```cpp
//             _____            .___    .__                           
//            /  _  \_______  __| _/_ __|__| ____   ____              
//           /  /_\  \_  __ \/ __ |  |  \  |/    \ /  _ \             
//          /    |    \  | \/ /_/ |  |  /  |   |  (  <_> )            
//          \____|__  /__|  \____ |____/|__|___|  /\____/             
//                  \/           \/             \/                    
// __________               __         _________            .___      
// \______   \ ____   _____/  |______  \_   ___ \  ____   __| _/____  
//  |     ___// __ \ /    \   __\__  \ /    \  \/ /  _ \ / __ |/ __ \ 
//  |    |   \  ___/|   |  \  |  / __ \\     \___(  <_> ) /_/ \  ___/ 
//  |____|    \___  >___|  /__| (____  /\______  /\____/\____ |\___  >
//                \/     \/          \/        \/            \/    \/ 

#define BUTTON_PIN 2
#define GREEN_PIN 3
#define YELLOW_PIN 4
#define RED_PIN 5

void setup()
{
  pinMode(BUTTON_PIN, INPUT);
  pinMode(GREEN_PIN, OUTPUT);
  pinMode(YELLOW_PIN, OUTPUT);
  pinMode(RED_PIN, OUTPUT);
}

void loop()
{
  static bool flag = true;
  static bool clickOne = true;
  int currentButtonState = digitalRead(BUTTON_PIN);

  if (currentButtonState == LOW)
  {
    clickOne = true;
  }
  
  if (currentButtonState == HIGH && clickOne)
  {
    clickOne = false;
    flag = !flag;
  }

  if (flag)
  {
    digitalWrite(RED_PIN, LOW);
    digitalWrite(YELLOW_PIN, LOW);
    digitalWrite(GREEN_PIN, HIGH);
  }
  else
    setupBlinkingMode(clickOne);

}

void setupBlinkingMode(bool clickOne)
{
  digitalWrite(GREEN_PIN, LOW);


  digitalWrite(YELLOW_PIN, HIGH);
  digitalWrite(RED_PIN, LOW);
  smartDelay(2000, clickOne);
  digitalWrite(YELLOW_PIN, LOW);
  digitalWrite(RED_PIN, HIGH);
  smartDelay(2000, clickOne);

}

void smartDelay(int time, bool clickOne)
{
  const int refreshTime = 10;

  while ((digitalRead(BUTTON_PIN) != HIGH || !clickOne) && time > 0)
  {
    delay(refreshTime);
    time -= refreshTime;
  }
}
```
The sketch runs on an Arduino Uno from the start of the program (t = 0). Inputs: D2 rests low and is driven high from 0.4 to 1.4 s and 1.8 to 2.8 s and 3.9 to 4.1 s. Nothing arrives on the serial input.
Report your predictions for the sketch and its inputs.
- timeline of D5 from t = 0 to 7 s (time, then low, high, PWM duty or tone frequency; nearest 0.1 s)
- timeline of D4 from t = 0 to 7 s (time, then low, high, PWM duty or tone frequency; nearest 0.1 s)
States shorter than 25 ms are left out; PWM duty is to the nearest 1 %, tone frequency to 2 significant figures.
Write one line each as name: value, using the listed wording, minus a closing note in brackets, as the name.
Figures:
timeline of D5 from t = 0 to 7 s: 0 s low; 2.4 s high; 4.4 s low; 6.4 s high
timeline of D4 from t = 0 to 7 s: 0 s low; 0.4 s high; 2.4 s low; 4.4 s high; 6.4 s low
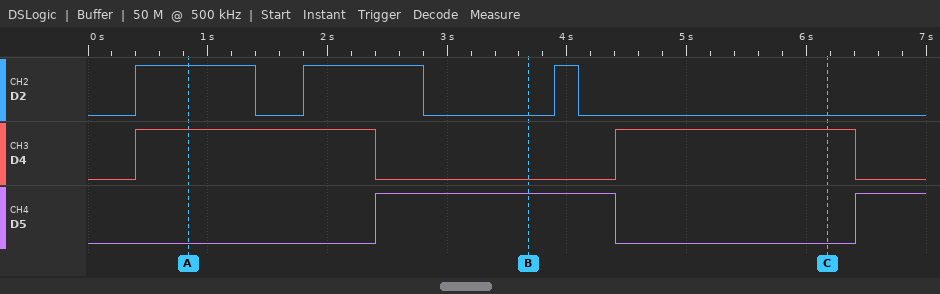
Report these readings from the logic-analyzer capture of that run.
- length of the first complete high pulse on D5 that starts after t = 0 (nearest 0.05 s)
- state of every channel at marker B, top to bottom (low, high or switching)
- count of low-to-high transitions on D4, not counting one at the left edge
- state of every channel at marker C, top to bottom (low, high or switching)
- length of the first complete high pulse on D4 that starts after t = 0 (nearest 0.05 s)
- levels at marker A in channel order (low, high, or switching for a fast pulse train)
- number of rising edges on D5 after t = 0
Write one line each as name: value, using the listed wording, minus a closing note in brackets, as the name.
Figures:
length of the first complete high pulse on D5 that starts after t = 0: 2.00 s
state of every channel at marker B, top to bottom: D2 low, D4 low, D5 high
count of low-to-high transitions on D4, not counting one at the left edge: 2
state of every channel at marker C, top to bottom: D2 low, D4 high, D5 low
length of the first complete high pulse on D4 that starts after t = 0: 2.00 s
levels at marker A in channel order: D2 high, D4 high, D5 low
number of rising edges on D5 after t = 0: 2
